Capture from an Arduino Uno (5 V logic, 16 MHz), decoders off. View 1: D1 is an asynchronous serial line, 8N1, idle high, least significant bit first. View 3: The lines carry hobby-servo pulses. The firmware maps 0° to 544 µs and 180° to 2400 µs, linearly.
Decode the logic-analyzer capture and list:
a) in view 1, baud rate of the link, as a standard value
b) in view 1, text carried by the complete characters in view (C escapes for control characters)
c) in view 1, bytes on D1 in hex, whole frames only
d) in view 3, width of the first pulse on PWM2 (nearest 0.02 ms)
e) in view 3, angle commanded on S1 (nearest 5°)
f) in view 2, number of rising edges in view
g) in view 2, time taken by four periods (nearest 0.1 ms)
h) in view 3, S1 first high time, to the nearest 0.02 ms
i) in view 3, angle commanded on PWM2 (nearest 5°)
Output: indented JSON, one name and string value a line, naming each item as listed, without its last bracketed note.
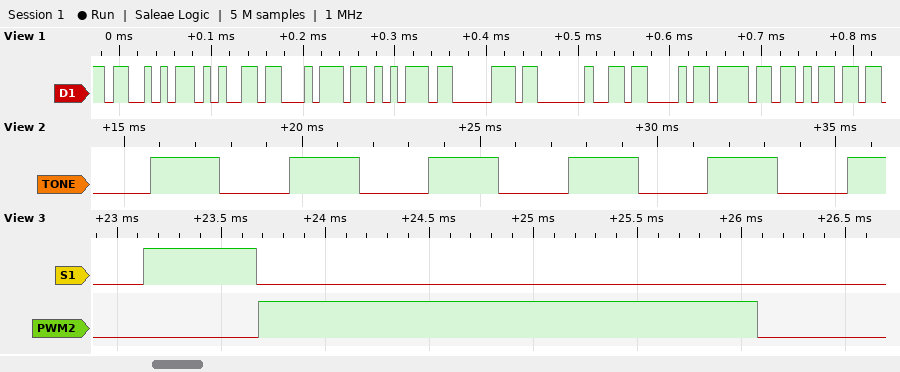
{
  "in view 1, baud rate of the link, as a standard value": "115200 baud",
  "in view 1, text carried by the complete characters in view": "\"Setup Com\"",
  "in view 1, bytes on D1 in hex, whole frames only": "53 65 74 75 70 20 43 6F 6D",
  "in view 3, width of the first pulse on PWM2": "2.40 ms",
  "in view 3, angle commanded on S1": "0°",
  "in view 2, number of rising edges in view": "6",
  "in view 2, time taken by four periods": "15.7 ms",
  "in view 3, S1 first high time, to the nearest 0.02 ms": "0.54 ms",
  "in view 3, angle commanded on PWM2": "180°"
}
